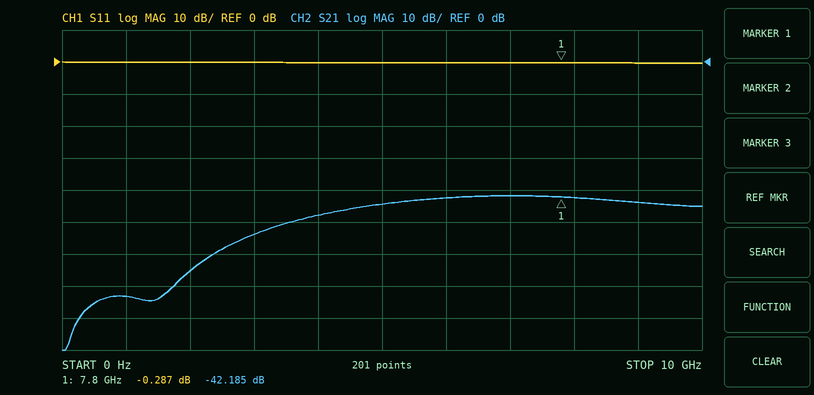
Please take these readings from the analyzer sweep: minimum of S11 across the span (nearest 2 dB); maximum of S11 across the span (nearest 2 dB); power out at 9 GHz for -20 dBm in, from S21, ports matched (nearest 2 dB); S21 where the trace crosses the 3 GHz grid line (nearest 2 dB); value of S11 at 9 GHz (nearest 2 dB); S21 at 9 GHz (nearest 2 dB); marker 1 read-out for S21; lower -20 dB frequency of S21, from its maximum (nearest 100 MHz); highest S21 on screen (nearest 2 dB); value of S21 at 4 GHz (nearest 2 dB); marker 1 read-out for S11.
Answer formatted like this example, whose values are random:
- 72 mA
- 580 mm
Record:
- 0 dB
- 0 dB
- -64 dBm
- -54 dB
- 0 dB
- -44 dB
- -42.185 dB
- 2.2 GHz
- -42 dB
- -48 dB
- -0.287 dB
